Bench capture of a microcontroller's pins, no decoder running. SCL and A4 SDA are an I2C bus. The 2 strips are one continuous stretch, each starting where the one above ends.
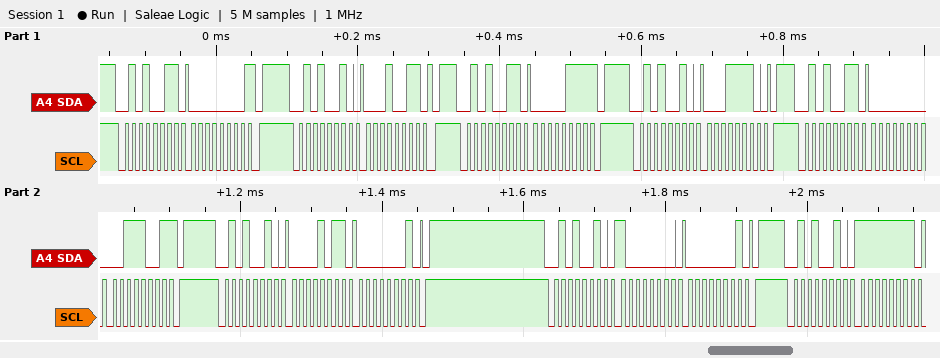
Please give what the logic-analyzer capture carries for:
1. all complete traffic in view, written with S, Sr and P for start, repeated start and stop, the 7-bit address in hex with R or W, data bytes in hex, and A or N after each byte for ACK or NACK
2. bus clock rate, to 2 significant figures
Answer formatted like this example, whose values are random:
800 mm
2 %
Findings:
S 29R A 00 N P S 29W A 13 A P S 29R A 07 N P S 29W A 1E A P S 29R A 00 A 39 N P S 29W A 0B A 01 A P S 29W A 80 A 01 A P S 29W A FF A
100 kHz
